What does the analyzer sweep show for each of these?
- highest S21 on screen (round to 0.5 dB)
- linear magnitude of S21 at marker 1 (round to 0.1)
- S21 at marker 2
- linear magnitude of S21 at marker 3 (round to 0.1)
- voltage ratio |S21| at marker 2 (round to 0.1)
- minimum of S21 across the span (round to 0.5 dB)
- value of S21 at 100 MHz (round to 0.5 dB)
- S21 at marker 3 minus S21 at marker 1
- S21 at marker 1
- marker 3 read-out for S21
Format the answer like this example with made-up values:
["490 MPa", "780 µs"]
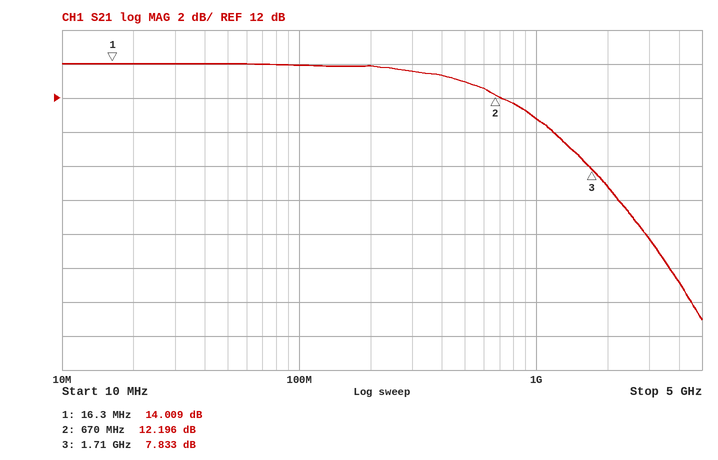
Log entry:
["14.0 dB", "5.0", "12.196 dB", "2.5", "4.1", "-1.0 dB", "14.0 dB", "-6.176 dB", "14.009 dB", "7.833 dB"]
